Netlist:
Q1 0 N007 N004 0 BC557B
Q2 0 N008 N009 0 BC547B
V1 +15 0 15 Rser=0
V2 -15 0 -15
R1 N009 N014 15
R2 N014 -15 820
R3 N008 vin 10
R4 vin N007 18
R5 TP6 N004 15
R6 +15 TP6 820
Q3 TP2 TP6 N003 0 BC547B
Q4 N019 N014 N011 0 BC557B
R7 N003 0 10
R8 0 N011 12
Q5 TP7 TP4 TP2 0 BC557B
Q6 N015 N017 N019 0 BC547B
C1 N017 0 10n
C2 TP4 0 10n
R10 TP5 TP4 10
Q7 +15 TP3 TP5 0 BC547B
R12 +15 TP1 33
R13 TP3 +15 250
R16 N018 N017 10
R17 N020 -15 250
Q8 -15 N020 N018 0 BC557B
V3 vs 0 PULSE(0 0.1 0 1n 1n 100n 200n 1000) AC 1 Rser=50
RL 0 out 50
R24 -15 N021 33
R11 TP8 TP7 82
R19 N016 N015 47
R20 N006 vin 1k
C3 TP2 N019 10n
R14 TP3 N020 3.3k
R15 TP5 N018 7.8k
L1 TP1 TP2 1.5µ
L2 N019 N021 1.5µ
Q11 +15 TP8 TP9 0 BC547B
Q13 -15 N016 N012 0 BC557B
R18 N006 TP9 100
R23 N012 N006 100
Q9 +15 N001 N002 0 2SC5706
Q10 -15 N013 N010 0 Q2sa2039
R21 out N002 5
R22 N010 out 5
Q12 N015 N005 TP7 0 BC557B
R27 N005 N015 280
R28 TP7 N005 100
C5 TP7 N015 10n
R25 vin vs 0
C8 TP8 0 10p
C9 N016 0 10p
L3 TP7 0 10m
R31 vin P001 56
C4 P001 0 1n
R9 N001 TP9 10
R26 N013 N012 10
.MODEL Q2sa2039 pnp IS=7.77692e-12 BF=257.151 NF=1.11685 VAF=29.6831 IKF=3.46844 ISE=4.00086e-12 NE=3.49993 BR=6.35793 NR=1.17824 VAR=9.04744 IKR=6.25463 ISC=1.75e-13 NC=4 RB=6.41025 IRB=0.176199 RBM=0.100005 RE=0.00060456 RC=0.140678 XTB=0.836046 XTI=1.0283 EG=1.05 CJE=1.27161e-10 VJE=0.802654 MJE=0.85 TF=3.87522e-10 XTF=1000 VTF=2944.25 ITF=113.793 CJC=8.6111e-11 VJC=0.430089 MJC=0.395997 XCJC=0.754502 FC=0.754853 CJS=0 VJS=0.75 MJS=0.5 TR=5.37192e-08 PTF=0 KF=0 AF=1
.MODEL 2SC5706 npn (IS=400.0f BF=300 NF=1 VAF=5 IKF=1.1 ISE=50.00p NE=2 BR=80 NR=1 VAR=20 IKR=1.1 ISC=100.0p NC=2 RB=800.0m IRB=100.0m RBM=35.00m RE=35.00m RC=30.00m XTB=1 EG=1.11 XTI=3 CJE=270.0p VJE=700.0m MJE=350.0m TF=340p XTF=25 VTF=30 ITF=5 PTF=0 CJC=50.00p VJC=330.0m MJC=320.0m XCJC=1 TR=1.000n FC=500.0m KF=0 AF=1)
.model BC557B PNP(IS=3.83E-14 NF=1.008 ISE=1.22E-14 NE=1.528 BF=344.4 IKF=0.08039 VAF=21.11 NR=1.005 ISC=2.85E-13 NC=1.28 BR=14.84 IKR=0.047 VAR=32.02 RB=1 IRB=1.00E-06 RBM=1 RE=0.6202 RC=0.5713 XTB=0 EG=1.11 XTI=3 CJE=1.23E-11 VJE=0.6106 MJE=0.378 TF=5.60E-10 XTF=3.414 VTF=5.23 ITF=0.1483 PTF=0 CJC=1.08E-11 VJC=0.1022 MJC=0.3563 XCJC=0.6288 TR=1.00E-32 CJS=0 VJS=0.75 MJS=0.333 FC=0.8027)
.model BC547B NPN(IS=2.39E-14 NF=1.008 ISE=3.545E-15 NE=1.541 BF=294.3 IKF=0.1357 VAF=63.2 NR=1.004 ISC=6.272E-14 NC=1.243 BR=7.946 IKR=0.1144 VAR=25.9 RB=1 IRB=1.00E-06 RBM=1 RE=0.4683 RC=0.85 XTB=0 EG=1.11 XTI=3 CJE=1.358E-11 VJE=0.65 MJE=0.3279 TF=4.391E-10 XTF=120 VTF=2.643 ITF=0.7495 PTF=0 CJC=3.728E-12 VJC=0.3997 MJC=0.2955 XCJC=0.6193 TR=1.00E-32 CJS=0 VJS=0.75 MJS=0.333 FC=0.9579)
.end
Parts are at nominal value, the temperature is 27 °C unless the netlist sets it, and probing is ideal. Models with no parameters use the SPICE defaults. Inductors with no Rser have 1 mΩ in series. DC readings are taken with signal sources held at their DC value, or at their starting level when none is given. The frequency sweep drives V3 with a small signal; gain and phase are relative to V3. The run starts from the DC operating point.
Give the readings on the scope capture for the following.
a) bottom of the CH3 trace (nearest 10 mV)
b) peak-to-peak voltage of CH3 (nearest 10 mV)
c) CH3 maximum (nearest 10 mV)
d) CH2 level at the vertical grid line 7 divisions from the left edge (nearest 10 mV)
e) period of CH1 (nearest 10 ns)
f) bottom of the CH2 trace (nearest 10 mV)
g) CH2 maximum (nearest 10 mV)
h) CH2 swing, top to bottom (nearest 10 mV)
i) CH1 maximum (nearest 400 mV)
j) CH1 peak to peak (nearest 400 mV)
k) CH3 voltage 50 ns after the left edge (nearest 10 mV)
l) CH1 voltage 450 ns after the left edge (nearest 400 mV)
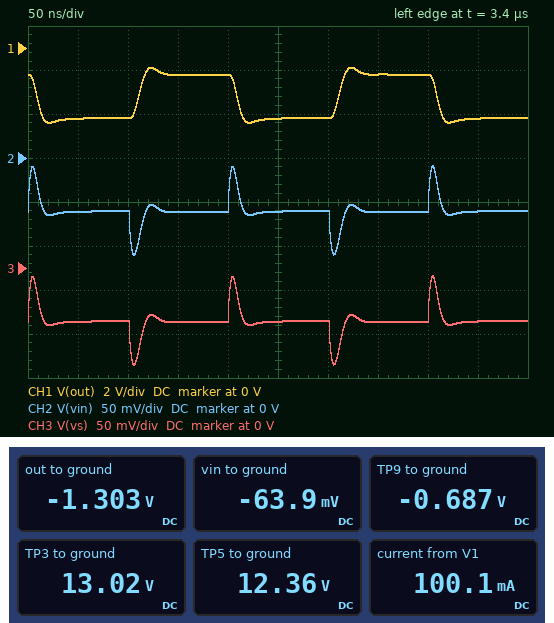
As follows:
-110 mV
100 mV
-10 mV
-60 mV
200 ns
-110 mV
-10 mV
100 mV
-800 mV
2.4 V
-60 mV
-3.2 V
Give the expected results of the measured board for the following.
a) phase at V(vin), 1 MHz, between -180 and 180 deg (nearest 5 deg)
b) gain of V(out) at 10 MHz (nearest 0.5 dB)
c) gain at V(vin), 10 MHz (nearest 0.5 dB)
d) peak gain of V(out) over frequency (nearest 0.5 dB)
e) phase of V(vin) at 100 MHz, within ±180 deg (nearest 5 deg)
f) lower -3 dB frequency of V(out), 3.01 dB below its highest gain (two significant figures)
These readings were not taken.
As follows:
70 deg
26.5 dB
-11.5 dB
26.5 dB
-40 deg
3.0 kHz
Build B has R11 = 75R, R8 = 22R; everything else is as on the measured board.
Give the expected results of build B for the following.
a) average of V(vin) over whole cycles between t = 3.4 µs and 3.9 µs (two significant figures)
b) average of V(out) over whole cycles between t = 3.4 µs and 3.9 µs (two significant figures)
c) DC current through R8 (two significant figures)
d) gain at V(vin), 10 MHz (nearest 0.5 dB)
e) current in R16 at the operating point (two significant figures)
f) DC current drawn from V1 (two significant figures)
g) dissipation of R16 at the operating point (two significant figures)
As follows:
-62 mV
-2.3 V
16 mA
-10.0 dB
160 µA
110 mA
250 nW
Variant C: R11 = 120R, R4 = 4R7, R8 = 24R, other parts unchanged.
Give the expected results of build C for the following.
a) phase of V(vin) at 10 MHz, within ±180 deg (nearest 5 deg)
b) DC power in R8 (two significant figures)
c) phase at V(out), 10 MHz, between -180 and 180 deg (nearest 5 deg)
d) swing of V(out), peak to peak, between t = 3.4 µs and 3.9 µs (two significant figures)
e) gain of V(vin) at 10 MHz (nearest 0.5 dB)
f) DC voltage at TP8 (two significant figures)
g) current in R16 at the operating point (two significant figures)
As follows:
65 deg
5.1 mW
145 deg
2.2 V
-9.5 dB
-2.4 mV
160 µA
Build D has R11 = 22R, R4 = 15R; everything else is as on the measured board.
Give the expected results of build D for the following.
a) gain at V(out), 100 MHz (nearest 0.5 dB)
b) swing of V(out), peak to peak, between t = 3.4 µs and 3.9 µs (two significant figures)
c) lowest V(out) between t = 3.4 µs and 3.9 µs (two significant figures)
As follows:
2.5 dB
2.6 V
-3.5 V
